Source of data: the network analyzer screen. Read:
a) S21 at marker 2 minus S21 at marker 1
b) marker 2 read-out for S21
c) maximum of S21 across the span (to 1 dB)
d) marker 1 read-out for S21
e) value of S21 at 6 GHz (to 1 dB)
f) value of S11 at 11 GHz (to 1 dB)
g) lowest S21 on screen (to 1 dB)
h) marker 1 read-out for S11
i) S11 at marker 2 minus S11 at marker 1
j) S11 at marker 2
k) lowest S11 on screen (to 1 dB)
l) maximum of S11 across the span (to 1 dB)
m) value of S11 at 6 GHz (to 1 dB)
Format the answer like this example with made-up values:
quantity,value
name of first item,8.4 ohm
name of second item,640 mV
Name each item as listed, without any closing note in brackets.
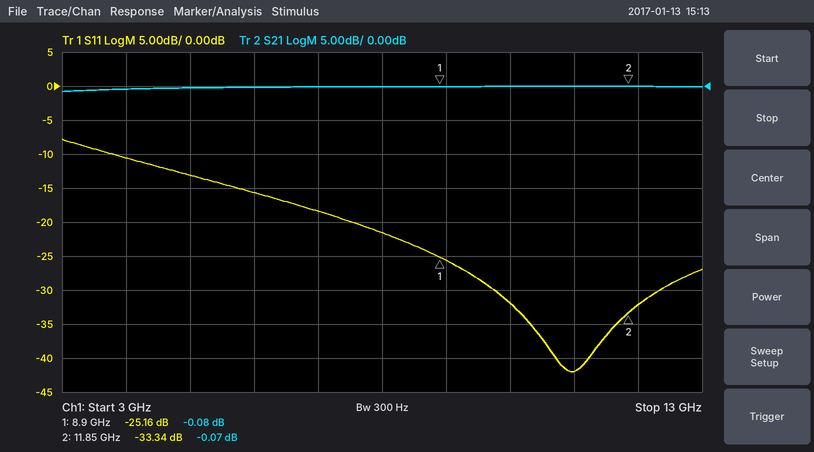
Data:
quantity,value
S21 at marker 2 minus S21 at marker 1,0.01 dB
marker 2 read-out for S21,-0.07 dB
maximum of S21 across the span,0 dB
marker 1 read-out for S21,-0.08 dB
value of S21 at 6 GHz,0 dB
value of S11 at 11 GHz,-42 dB
lowest S21 on screen,-1 dB
marker 1 read-out for S11,-25.16 dB
S11 at marker 2 minus S11 at marker 1,-8.18 dB
S11 at marker 2,-33.34 dB
lowest S11 on screen,-42 dB
maximum of S11 across the span,-8 dB
value of S11 at 6 GHz,-16 dB
